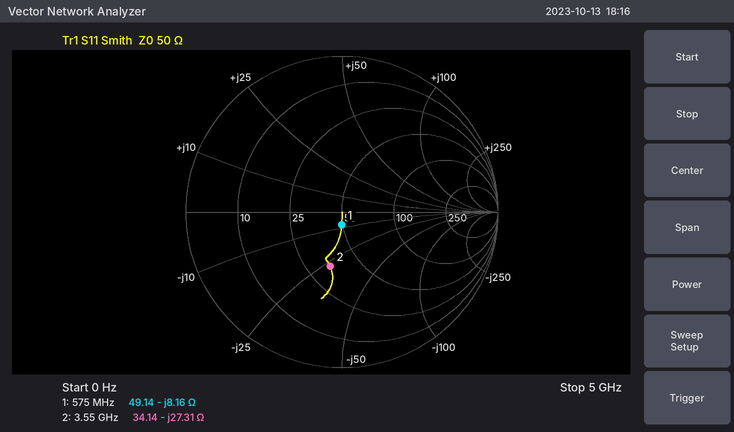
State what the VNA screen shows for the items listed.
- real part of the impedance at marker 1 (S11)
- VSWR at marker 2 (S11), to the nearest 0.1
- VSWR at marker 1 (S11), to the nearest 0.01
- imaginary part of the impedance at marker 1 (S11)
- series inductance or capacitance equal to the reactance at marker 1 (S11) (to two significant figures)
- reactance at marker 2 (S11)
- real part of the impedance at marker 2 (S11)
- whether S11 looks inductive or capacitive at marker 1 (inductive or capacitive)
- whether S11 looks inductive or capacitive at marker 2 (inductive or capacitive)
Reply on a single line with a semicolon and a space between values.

49.14 Ω; 2.1; 1.18; -8.16 Ω; 34 pF; -27.31 Ω; 34.14 Ω; capacitive; capacitive
